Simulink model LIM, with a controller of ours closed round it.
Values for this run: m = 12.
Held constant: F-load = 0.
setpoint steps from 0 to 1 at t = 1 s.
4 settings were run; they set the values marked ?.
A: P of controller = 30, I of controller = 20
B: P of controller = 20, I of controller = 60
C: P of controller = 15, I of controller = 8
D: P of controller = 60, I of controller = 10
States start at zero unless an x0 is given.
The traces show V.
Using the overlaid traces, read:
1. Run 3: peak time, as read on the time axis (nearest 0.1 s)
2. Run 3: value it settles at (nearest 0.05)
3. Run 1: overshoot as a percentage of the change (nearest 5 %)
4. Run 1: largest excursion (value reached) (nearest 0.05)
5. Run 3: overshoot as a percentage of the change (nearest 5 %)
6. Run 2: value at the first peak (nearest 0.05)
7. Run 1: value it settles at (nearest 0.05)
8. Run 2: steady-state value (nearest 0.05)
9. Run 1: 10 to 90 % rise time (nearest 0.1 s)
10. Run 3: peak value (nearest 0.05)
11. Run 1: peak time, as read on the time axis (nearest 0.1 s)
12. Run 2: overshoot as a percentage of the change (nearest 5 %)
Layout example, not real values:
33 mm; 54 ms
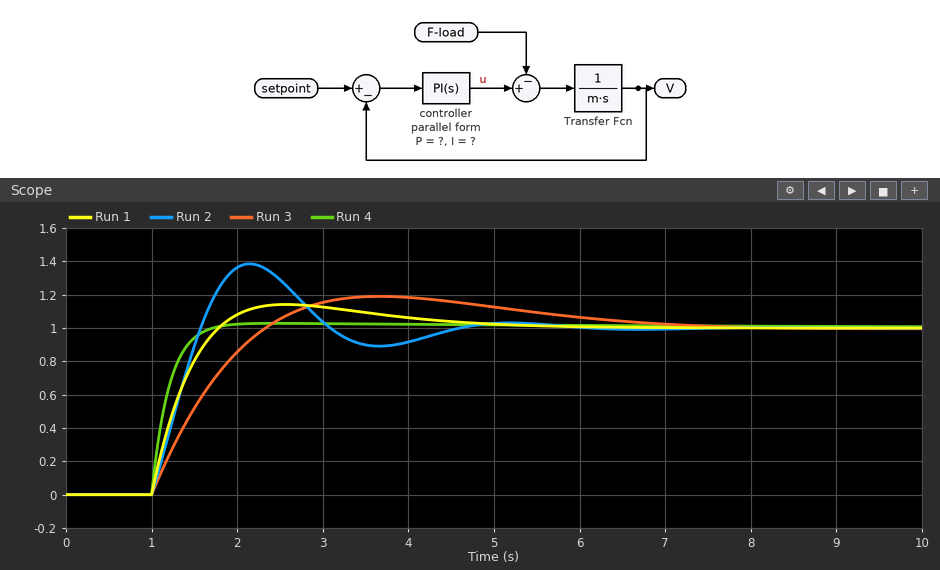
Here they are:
3.7 s; 1.00; 15 %; 1.15; 20 %; 1.40; 1.00; 1.00; 0.6 s; 1.20; 2.6 s; 40 %
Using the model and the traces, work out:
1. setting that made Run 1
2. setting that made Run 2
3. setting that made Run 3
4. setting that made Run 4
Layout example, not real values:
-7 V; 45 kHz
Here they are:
A; B; C; D
